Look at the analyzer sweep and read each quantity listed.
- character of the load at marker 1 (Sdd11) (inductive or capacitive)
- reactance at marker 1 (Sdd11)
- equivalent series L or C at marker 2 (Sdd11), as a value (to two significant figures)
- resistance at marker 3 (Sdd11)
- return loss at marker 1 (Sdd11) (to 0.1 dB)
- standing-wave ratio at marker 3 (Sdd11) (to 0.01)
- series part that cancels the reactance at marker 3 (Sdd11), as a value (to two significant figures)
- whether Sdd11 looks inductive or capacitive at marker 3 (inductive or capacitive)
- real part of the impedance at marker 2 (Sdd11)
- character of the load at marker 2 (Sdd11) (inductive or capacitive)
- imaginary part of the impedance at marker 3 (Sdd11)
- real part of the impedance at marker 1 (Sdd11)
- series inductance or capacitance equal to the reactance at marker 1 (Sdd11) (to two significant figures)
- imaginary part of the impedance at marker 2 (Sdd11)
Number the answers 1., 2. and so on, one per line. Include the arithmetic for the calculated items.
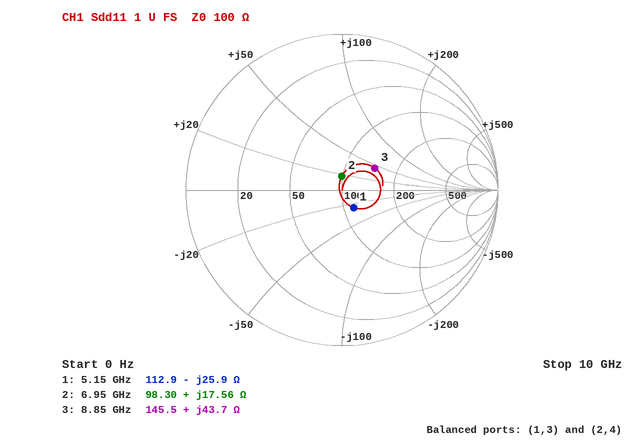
1. capacitive
2. -25.9 Ω
3. L = 17.56 Ω/(2π × 6.95 GHz) ≈ 402 pH, so 400 pH to two significant figures
4. 145.5 Ω
5. 17.4 dB
6. 1.68
7. C = 1/(2π × 8.85 GHz × 43.7 Ω) ≈ 412 fF, so 410 fF to two significant figures
8. inductive
9. 98.30 Ω
10. inductive
11. +43.7 Ω
12. 112.9 Ω
13. C = 1/(2π × 5.15 GHz × 25.9 Ω) ≈ 1.2 pF
14. +17.56 Ω
